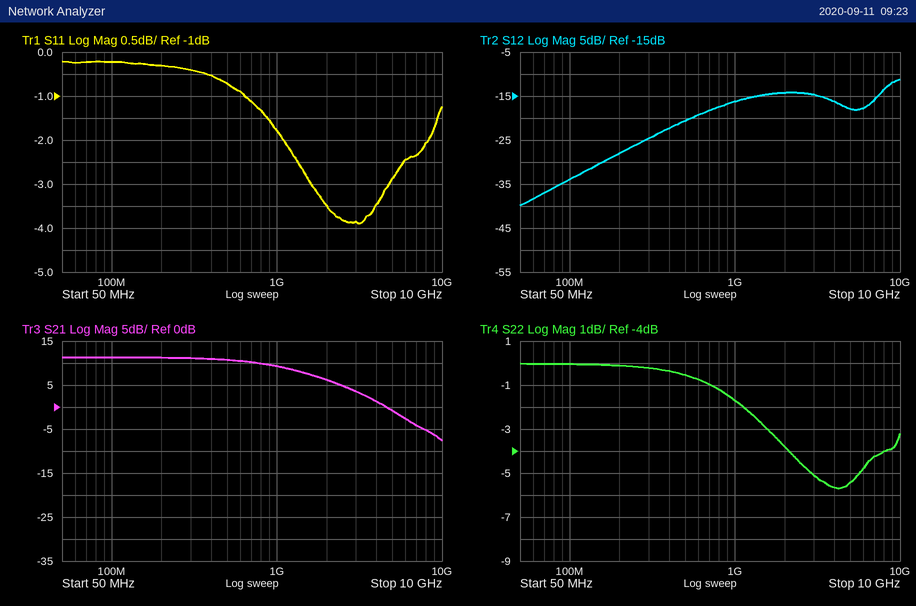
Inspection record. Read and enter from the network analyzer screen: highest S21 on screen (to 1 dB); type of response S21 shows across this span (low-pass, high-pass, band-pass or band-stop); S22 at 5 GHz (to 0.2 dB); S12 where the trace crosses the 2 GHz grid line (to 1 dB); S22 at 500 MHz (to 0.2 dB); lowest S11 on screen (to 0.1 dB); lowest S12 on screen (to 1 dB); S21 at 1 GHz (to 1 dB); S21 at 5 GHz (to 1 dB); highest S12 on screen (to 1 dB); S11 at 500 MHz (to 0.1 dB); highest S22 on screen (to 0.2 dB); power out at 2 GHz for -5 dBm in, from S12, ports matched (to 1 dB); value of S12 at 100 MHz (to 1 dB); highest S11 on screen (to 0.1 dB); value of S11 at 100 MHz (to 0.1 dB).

11 dB
low-pass
-5.4 dB
-14 dB
-0.6 dB
-3.9 dB
-40 dB
9 dB
-1 dB
-11 dB
-0.7 dB
0.0 dB
-19 dBm
-34 dB
-0.2 dB
-0.2 dB
